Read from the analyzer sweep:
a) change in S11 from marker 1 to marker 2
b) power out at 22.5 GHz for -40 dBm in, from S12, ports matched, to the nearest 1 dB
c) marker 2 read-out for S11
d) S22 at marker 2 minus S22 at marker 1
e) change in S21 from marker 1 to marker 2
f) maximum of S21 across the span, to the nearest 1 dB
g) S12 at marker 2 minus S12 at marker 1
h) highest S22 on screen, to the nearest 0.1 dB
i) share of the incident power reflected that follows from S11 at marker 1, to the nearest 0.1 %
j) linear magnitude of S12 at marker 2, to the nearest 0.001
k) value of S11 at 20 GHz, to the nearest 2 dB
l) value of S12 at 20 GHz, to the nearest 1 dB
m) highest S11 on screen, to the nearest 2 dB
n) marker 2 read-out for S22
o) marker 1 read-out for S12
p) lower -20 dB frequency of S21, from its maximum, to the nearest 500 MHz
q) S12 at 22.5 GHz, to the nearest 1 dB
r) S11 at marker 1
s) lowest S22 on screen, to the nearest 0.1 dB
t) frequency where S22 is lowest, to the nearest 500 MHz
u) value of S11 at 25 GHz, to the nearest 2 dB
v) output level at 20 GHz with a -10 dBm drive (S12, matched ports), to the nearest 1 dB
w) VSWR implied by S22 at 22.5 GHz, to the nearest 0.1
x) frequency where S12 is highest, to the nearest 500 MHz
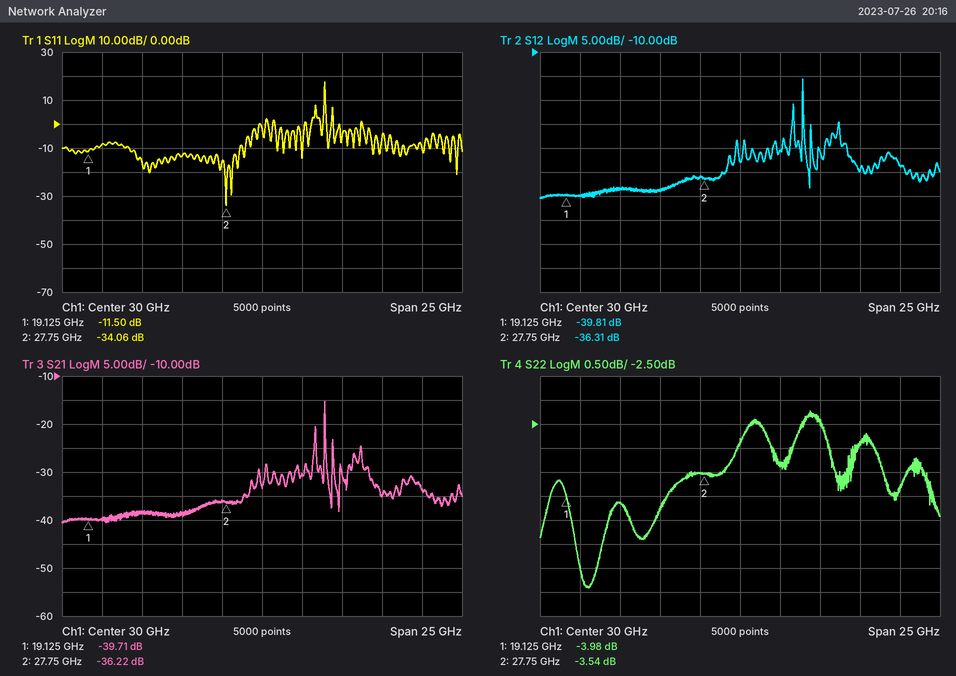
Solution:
-22.56 dB
-78 dBm
-34.06 dB
0.44 dB
3.49 dB
-15 dB
3.50 dB
-2.2 dB
7.1 %
0.015
-8 dB
-40 dB
18 dB
-3.54 dB
-39.81 dB
29.0 GHz
-38 dB
-11.50 dB
-5.9 dB
20.5 GHz
-14 dB
-50 dBm
4.3
34.0 GHz
